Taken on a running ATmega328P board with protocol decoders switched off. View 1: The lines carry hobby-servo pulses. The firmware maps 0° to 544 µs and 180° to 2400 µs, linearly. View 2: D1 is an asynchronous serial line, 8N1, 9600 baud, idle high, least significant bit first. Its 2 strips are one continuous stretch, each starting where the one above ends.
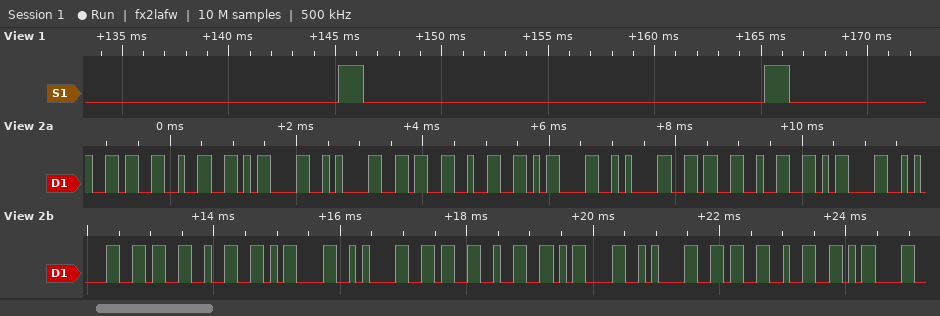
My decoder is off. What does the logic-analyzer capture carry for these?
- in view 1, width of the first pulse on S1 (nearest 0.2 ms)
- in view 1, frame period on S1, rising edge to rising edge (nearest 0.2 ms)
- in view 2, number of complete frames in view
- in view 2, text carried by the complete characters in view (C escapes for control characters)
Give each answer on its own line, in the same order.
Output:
1.2 ms
20.0 ms
23
"62\r\n62\r\n62\r\n62\r\n62\r\n62\r"
